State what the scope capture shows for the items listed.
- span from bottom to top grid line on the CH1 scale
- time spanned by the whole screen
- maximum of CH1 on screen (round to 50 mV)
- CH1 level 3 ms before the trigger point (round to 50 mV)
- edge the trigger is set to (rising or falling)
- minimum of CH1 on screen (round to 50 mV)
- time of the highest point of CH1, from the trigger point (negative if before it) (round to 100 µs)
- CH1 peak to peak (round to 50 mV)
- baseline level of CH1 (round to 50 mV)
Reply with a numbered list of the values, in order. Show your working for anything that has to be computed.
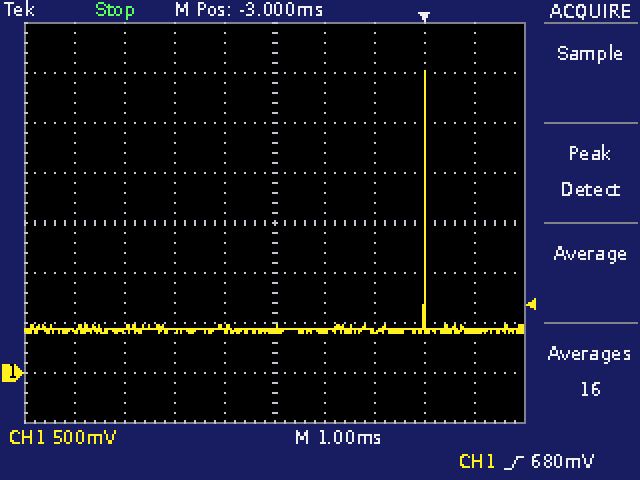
1. 4 V
2. 10 ms
3. 3.00 V
4. 450 mV
5. rising
6. 400 mV
7. 0.0 ms
8. 3.00 V − (400 mV) = 2.60 V
9. 450 mV
